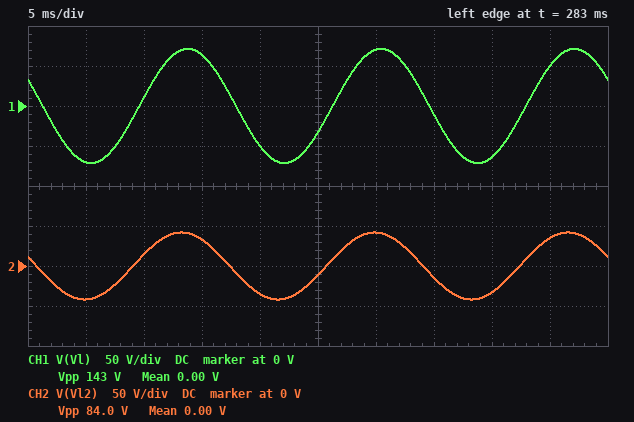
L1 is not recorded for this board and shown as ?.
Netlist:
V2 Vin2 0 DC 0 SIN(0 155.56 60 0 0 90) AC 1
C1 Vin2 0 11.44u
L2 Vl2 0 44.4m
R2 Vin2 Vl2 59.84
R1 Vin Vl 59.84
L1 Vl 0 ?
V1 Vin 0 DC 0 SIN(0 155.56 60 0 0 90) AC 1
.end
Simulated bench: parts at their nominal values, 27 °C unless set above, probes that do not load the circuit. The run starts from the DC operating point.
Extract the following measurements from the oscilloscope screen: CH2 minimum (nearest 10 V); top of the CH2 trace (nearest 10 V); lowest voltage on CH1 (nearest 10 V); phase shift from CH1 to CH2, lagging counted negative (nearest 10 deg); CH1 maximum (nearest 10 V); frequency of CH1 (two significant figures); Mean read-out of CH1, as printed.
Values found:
-40 V
40 V
-70 V
10 deg
70 V
60 Hz
0.00 V
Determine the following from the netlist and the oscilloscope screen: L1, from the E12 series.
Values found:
82 mH
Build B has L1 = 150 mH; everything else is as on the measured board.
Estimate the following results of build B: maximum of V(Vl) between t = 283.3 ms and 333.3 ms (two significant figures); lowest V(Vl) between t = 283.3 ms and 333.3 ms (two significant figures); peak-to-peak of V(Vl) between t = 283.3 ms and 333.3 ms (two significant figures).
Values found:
110 V
-110 V
210 V
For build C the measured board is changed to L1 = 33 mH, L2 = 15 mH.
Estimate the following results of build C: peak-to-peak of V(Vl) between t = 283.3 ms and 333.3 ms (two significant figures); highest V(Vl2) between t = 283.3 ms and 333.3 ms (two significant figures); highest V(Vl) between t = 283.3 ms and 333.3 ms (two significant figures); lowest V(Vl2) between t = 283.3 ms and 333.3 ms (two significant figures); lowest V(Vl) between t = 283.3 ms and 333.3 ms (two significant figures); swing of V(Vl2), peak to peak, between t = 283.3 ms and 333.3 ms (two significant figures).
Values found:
63 V
15 V
32 V
-15 V
-32 V
29 V
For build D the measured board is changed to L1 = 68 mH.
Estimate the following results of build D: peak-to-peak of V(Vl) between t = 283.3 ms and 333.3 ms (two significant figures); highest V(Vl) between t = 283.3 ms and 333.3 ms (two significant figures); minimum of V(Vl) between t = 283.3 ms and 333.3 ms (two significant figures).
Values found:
120 V
61 V
-61 V
